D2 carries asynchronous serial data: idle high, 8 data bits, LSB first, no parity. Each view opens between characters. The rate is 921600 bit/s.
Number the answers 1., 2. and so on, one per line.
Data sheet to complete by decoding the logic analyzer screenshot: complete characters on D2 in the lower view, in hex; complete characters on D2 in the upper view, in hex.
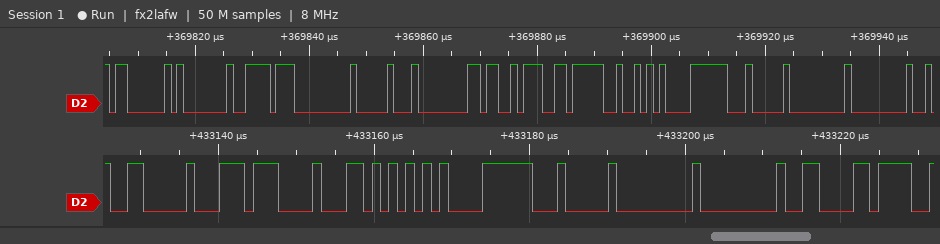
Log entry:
1. 06, DC, 88, 55, F8, 04, 00, 00, 86
2. 03, 01, DE, 00, 10, 80, D3, F6, 52, F8, 04, 00, 00
